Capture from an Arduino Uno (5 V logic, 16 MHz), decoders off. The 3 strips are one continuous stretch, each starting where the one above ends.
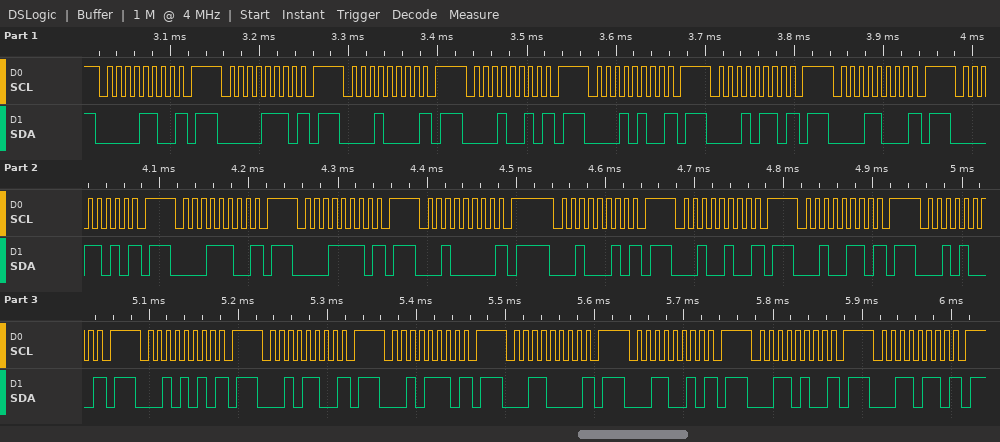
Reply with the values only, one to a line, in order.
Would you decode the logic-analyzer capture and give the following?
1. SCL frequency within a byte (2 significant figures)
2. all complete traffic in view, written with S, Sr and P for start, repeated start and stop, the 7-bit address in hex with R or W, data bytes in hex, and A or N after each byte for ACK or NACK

100 kHz
S 06W N P S 07W N P S 08W N P S 09W N P S 0AW N P S 0BW N P S 0CW N P S 0DW N P S 0EW N P S 0FW N P S 10W N P S 11W N P S 12W N P S 13W N P S 14W N P S 15W N P S 16W N P S 17W N P S 18W N P S 19W N P S 1AW N P S 1BW N P
